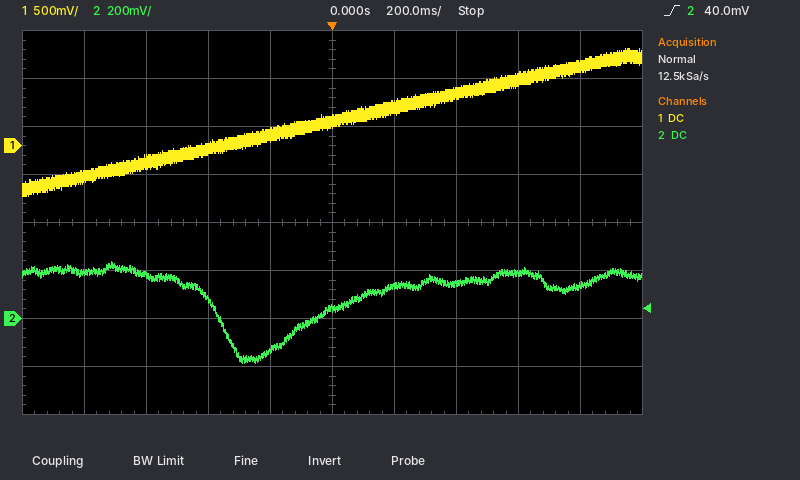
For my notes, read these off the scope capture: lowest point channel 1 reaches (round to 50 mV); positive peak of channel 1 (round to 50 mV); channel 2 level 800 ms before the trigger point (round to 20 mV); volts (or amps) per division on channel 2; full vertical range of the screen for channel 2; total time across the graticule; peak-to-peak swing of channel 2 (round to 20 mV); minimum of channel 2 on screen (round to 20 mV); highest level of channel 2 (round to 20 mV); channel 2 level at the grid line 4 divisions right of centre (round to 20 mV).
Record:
-500 mV
1.00 V
200 mV
200 mV
1.6 V
2 s
420 mV
-180 mV
240 mV
140 mV
